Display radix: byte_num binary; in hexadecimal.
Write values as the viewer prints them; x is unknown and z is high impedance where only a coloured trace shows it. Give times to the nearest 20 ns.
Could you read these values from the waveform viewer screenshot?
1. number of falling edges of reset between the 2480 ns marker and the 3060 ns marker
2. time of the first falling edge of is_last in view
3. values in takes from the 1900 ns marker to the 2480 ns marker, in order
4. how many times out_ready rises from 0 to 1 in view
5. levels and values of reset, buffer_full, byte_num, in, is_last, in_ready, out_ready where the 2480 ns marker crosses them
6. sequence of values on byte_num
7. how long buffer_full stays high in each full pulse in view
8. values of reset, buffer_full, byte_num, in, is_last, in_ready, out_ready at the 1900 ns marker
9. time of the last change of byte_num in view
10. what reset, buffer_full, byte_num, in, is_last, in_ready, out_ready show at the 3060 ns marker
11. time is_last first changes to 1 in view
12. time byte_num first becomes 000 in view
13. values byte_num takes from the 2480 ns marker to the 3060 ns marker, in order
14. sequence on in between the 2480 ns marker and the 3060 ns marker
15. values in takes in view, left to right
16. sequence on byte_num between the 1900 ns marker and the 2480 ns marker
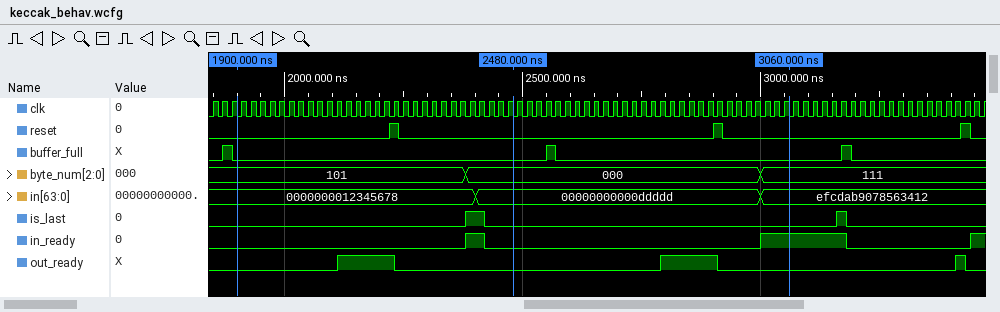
1
2420 ns
0000000012345678, 00000000000ddddd
3
reset=0, buffer_full=0, byte_num=000, in=00000000000ddddd, is_last=0, in_ready=0, out_ready=0
101, 000, 111
20 ns, 20 ns, 20 ns
reset=0, buffer_full=0, byte_num=101, in=0000000012345678, is_last=0, in_ready=0, out_ready=0
3000 ns
reset=0, buffer_full=0, byte_num=111, in=efcdab9078563412, is_last=0, in_ready=1, out_ready=0
2380 ns
2380 ns
000, 111
00000000000ddddd, efcdab9078563412
0000000012345678, 00000000000ddddd, efcdab9078563412
101, 000
